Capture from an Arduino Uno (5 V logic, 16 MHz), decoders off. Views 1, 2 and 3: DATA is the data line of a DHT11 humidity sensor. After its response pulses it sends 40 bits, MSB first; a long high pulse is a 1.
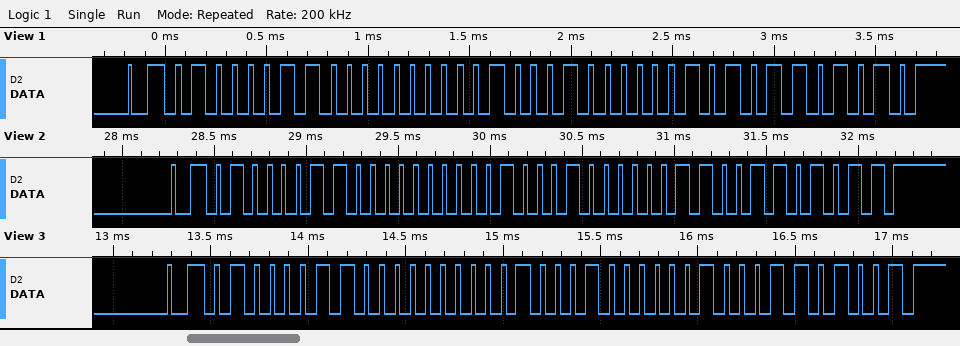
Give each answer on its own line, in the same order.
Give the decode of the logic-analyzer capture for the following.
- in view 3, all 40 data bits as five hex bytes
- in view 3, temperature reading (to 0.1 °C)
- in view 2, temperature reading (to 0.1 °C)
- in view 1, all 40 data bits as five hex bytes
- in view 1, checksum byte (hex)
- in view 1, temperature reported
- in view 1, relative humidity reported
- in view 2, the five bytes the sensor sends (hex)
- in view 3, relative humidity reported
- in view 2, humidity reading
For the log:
43 00 22 04 69
34.4 °C
34.6 °C
43 00 22 05 6A
0x6A
34.5 °C
67 %
43 00 22 06 6B
67 %
67 %
